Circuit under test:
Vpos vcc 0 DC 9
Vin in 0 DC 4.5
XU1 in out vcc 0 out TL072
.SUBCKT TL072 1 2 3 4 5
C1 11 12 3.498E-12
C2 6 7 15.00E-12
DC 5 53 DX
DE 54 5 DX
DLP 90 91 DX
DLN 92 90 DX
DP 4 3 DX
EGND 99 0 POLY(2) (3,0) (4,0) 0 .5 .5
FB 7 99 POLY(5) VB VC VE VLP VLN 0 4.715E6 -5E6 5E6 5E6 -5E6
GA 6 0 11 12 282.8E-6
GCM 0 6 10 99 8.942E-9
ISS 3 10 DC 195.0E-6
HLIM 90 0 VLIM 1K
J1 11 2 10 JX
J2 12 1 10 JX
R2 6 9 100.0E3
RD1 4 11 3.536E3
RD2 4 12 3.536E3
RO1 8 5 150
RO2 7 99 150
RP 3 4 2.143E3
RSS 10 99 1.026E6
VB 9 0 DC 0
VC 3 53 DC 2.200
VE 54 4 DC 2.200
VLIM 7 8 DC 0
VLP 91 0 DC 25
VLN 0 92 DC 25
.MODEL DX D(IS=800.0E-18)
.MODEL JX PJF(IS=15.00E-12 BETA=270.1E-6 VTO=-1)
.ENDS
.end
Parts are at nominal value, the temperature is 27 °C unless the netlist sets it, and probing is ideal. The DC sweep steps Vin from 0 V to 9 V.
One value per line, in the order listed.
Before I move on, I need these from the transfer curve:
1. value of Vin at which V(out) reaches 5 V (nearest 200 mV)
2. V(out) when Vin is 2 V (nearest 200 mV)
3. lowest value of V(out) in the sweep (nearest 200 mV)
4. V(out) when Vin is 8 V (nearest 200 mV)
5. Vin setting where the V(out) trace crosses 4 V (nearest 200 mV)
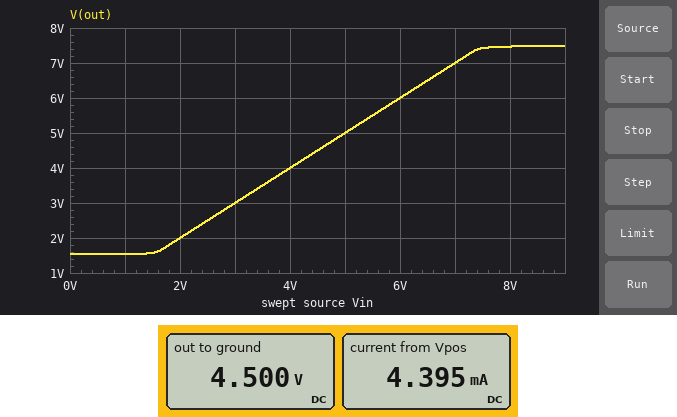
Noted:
5.0 V
2.0 V
1.6 V
7.4 V
4.0 V
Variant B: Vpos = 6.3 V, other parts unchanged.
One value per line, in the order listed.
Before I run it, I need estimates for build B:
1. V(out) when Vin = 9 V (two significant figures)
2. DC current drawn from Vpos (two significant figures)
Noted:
4.8 V
3.1 mA
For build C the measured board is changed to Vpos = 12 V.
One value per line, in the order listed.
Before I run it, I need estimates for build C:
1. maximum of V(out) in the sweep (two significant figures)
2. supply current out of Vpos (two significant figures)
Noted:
9.0 V
5.8 mA
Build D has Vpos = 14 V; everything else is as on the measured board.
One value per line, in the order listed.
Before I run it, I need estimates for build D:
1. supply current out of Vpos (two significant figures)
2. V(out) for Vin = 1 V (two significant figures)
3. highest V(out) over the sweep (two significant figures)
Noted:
6.7 mA
1.5 V
9.0 V
